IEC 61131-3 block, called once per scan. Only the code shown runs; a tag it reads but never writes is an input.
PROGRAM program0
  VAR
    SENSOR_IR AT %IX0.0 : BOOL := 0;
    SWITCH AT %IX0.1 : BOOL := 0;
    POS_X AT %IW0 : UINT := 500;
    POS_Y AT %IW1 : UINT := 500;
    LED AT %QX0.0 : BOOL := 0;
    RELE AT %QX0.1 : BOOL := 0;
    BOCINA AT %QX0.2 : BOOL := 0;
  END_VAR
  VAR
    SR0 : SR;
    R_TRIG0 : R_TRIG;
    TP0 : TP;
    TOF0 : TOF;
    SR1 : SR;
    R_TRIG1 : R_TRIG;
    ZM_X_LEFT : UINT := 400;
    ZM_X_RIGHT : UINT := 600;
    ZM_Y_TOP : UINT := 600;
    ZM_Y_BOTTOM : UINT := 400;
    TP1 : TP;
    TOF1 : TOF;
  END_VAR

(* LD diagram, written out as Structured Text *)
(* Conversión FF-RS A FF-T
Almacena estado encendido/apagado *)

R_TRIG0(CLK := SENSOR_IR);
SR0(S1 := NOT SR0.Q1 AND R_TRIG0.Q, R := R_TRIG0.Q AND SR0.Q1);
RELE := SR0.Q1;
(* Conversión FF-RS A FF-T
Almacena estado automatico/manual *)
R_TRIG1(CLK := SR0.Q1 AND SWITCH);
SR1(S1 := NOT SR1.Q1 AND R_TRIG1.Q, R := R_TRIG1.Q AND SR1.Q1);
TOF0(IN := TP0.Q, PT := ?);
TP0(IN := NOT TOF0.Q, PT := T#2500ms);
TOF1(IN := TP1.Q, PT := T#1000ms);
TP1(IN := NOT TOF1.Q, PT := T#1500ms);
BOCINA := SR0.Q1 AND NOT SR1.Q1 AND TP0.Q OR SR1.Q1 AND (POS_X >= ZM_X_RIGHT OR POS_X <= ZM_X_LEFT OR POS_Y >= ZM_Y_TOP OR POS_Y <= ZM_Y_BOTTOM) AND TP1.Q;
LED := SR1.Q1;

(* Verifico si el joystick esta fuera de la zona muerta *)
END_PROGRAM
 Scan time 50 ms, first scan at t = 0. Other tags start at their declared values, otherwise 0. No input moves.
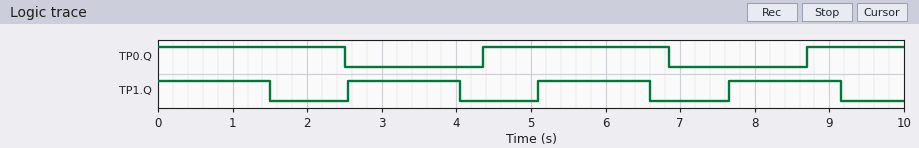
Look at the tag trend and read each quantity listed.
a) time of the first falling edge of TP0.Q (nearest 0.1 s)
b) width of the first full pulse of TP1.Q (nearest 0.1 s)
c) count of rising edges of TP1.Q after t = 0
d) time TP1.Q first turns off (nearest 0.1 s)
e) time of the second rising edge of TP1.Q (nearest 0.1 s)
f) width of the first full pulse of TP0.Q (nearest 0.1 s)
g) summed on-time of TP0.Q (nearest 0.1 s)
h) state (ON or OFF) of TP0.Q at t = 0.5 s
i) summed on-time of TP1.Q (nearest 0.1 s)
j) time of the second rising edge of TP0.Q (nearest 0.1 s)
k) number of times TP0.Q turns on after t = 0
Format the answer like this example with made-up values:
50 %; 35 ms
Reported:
2.5 s; 1.5 s; 3; 1.5 s; 5.1 s; 2.5 s; 6.3 s; ON; 6.0 s; 8.7 s; 2
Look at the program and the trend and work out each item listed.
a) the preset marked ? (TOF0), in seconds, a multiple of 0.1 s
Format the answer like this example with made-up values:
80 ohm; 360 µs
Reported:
1.8 s
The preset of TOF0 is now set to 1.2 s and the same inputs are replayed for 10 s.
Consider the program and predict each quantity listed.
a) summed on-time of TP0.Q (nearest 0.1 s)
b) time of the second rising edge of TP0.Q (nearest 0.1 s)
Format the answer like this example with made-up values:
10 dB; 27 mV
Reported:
7.5 s; 7.5 s
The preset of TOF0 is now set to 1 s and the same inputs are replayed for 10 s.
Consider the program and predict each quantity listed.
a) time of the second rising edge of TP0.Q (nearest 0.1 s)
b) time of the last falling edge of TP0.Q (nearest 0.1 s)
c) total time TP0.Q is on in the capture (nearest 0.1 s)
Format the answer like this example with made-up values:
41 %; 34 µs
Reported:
7.1 s; 9.6 s; 7.5 s
